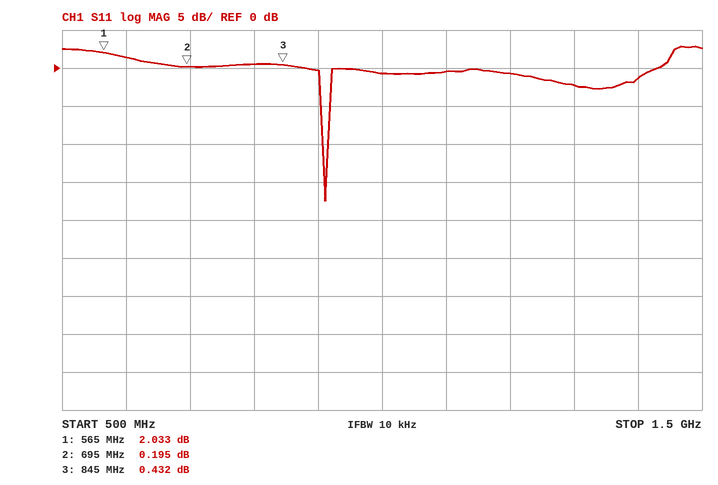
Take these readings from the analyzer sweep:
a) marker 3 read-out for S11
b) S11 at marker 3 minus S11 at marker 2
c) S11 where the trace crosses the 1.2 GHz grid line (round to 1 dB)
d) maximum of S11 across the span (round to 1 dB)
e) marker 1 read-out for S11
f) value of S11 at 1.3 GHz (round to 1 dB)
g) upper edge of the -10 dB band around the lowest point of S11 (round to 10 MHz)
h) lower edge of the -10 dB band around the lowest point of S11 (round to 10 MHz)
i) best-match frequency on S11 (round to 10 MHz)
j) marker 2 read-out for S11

0.432 dB
0.237 dB
-1 dB
3 dB
2.033 dB
-2 dB
920 MHz
910 MHz
910 MHz
0.195 dB
